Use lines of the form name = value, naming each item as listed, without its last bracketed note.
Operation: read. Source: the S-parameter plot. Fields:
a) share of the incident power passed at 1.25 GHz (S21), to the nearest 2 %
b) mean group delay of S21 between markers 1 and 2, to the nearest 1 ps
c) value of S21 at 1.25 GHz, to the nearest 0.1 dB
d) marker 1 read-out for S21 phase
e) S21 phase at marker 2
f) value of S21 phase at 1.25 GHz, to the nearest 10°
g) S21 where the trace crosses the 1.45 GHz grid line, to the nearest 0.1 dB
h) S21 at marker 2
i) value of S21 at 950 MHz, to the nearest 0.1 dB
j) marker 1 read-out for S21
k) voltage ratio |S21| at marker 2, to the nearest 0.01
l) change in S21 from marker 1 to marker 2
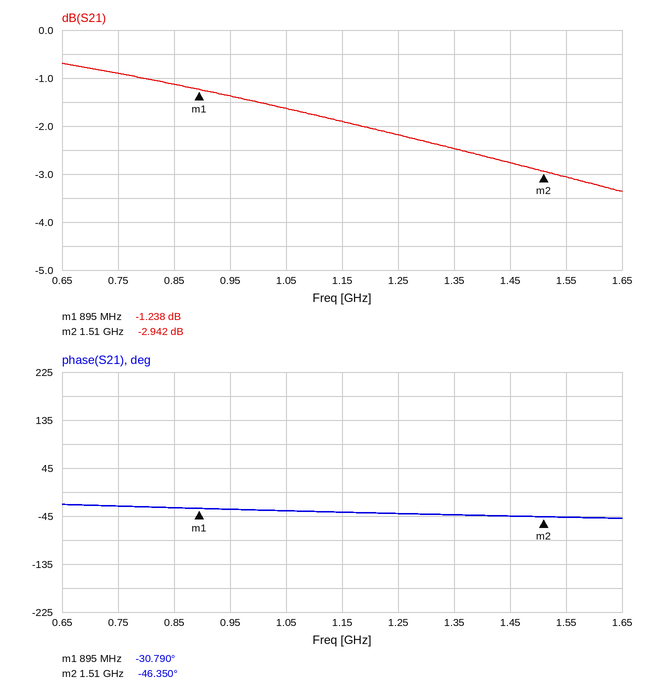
share of the incident power passed at 1.25 GHz (S21), to the nearest 2 % = 60 %
mean group delay of S21 between markers 1 and 2, to the nearest 1 ps = 70 ps
value of S21 at 1.25 GHz, to the nearest 0.1 dB = -2.2 dB
marker 1 read-out for S21 phase = -30.790°
S21 phase at marker 2 = -46.350°
value of S21 phase at 1.25 GHz, to the nearest 10° = -40°
S21 where the trace crosses the 1.45 GHz grid line, to the nearest 0.1 dB = -2.8 dB
S21 at marker 2 = -2.942 dB
value of S21 at 950 MHz, to the nearest 0.1 dB = -1.4 dB
marker 1 read-out for S21 = -1.238 dB
voltage ratio |S21| at marker 2, to the nearest 0.01 = 0.71
change in S21 from marker 1 to marker 2 = -1.704 dB
